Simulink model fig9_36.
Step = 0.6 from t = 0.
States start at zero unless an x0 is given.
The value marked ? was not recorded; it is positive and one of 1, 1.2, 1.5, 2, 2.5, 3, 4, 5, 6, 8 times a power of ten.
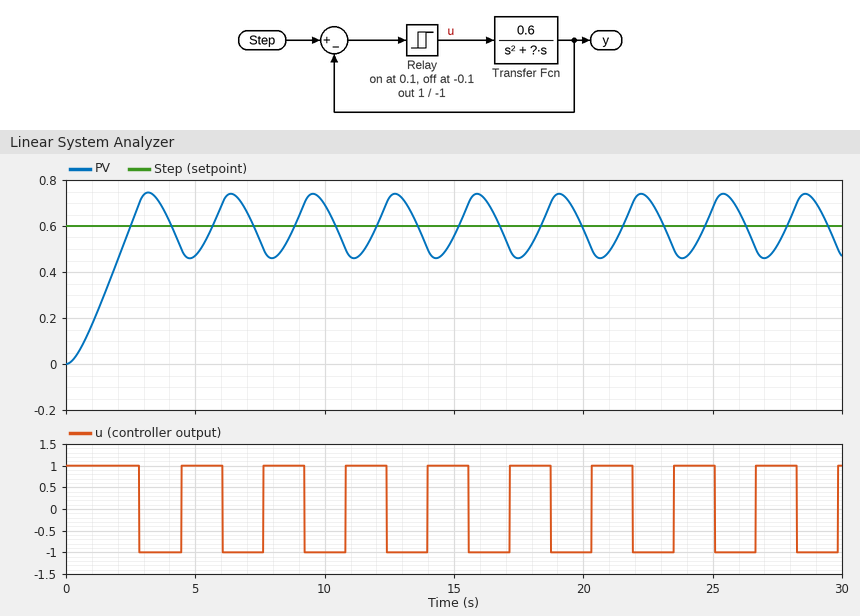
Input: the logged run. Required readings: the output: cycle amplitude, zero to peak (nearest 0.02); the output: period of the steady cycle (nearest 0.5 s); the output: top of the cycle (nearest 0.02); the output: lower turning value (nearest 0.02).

0.14
3.0 s
0.74
0.46
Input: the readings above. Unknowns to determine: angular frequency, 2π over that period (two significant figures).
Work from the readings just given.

2.1 rad/s
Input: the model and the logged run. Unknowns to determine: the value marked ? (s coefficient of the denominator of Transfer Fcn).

2
